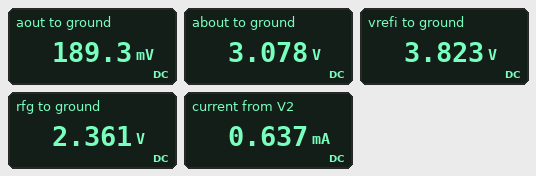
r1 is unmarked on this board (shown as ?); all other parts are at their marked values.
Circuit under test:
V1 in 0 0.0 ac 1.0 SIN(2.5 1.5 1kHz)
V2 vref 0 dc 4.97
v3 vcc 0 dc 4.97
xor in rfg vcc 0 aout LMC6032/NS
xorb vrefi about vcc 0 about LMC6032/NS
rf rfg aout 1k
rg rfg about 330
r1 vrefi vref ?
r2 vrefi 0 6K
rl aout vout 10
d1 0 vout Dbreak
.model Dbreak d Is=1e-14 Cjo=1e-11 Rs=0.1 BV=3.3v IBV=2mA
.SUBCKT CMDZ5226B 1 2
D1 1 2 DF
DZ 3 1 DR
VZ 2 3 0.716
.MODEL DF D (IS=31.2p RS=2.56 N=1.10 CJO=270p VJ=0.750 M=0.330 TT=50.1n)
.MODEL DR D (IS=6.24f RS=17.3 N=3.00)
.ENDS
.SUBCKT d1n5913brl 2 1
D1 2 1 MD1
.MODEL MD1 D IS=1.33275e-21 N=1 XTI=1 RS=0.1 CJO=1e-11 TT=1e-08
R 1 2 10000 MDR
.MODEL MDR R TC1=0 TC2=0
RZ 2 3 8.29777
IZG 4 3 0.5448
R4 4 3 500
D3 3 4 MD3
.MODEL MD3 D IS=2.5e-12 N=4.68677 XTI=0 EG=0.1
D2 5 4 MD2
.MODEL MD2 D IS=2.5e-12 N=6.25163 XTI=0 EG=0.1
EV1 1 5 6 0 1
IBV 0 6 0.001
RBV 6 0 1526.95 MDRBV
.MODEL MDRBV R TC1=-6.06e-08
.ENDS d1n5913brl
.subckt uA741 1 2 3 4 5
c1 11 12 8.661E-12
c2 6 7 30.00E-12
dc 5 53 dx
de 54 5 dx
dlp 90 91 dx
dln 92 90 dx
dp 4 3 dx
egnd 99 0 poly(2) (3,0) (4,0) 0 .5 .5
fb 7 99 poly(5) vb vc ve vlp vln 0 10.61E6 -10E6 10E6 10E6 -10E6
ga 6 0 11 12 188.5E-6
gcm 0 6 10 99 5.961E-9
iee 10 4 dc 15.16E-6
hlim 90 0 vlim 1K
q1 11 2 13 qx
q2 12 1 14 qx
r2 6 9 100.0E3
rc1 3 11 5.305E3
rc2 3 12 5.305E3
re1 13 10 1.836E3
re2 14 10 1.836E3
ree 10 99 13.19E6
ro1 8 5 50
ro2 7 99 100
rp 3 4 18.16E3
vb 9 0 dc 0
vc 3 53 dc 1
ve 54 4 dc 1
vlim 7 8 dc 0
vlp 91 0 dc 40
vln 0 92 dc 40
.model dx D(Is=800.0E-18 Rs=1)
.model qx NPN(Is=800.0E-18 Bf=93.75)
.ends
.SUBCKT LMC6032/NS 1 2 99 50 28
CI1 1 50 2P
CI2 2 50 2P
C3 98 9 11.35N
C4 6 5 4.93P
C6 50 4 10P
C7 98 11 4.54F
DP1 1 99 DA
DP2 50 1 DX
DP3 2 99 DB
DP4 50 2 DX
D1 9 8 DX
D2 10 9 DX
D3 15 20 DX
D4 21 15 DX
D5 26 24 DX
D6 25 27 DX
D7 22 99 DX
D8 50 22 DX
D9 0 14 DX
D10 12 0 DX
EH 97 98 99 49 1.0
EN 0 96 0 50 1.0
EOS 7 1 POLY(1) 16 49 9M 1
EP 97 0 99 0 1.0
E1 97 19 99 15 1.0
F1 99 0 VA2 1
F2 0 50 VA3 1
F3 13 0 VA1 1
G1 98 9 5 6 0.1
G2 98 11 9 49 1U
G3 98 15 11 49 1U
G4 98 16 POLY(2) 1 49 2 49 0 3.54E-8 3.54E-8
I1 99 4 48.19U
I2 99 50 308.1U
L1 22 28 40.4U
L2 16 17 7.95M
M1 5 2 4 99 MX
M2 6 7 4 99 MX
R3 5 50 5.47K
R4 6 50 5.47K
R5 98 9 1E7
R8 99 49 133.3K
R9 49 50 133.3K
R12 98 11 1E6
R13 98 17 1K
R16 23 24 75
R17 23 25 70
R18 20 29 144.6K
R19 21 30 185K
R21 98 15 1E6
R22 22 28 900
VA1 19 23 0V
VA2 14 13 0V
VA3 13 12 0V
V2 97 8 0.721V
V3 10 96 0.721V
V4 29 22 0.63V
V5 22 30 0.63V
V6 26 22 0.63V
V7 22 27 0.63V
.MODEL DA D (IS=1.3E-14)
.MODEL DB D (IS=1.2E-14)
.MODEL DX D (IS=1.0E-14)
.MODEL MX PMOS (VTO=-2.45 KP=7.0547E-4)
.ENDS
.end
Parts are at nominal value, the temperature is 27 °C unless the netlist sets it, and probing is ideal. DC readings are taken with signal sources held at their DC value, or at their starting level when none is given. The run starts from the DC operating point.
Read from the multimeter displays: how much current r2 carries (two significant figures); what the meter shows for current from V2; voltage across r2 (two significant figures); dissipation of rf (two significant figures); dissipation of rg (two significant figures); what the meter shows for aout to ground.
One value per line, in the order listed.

640 µA
0.637 mA
3.8 V
4.7 mW
1.6 mW
189.3 mV
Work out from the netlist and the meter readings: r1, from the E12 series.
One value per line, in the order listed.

1.8 kΩ
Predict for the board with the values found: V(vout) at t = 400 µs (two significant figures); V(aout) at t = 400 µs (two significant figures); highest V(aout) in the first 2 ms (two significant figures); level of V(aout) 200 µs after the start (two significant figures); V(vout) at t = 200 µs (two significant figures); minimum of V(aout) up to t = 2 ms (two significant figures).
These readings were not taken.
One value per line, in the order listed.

2.7 V
2.7 V
2.7 V
2.7 V
2.7 V
190 mV
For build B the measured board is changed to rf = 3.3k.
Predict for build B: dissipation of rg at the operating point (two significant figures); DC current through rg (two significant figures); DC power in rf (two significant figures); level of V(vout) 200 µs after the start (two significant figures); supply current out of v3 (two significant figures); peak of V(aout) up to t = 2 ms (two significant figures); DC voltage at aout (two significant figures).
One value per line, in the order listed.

230 µW
830 µA
2.3 mW
2.4 V
1.5 mA
2.5 V
65 mV
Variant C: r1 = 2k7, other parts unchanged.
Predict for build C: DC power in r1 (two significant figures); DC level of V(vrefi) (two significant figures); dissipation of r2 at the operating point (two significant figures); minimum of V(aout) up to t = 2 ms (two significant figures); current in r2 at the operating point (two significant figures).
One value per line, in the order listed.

880 µW
3.4 V
2.0 mW
190 mV
570 µA
